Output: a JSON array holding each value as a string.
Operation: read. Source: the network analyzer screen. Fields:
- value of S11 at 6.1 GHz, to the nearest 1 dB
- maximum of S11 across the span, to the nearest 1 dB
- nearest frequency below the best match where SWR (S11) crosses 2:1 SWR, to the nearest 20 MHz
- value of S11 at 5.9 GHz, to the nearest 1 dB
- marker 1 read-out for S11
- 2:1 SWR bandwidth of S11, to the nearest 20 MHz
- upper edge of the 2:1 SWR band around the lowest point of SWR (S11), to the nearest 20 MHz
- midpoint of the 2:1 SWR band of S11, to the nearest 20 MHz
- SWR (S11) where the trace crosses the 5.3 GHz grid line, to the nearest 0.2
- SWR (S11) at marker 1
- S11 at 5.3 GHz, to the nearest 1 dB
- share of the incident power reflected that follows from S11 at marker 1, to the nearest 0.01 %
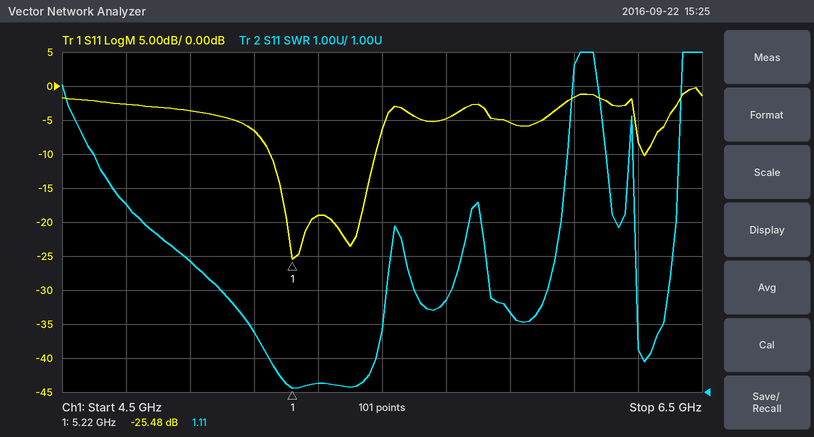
["-2 dB", "0 dB", "5.14 GHz", "-5 dB", "-25.48 dB", "340 MHz", "5.48 GHz", "5.32 GHz", "1.2", "1.11", "-19 dB", "0.28 %"]
